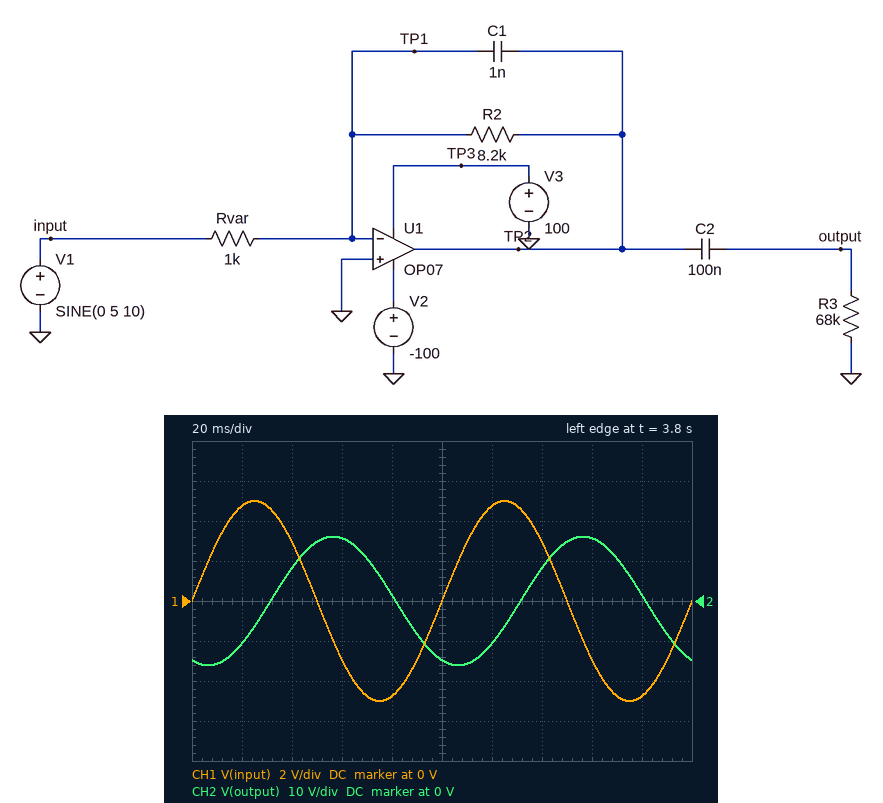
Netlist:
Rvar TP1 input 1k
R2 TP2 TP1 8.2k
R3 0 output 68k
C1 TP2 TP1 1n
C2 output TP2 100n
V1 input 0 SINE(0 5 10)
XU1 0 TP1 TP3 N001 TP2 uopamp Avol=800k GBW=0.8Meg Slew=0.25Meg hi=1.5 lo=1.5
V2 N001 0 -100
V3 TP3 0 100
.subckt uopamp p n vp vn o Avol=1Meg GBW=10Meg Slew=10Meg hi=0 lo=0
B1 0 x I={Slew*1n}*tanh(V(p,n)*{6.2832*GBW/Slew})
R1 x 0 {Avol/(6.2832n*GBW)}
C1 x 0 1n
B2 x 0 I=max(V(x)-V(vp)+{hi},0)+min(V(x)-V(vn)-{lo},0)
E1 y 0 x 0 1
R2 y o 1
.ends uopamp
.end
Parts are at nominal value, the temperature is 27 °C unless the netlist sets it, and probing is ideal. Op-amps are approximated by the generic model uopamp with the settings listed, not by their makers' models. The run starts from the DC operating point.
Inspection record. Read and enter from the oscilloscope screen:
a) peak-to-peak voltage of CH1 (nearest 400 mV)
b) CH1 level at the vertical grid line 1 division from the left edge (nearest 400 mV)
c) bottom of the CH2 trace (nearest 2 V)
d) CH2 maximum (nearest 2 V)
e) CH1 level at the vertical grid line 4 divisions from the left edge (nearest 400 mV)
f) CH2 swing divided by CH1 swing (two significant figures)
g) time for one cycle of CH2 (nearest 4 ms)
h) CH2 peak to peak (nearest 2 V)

10.0 V
4.8 V
-16 V
16 V
-4.8 V
3.2
100 ms
32 V
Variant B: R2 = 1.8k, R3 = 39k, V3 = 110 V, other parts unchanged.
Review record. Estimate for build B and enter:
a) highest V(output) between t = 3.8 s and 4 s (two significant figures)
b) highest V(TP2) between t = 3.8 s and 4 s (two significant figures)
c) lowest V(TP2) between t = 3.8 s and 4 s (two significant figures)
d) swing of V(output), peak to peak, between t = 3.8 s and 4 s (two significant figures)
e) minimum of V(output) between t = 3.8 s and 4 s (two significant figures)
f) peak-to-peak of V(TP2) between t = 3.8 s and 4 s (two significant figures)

2.1 V
9.0 V
-9.0 V
4.3 V
-2.1 V
18 V
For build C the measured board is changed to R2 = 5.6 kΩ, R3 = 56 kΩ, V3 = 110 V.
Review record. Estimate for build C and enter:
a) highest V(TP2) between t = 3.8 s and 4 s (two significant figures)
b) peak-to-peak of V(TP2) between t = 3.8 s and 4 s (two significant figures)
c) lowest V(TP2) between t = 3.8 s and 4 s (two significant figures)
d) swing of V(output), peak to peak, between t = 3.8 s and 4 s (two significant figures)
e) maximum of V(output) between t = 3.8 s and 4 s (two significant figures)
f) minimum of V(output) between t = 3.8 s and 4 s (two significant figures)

28 V
56 V
-28 V
19 V
9.3 V
-9.3 V
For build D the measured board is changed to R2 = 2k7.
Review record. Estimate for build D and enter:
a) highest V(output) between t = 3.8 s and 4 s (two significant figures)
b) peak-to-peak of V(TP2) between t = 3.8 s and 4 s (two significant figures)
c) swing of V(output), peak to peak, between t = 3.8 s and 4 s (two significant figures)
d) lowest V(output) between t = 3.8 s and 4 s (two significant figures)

5.3 V
27 V
11 V
-5.3 V
